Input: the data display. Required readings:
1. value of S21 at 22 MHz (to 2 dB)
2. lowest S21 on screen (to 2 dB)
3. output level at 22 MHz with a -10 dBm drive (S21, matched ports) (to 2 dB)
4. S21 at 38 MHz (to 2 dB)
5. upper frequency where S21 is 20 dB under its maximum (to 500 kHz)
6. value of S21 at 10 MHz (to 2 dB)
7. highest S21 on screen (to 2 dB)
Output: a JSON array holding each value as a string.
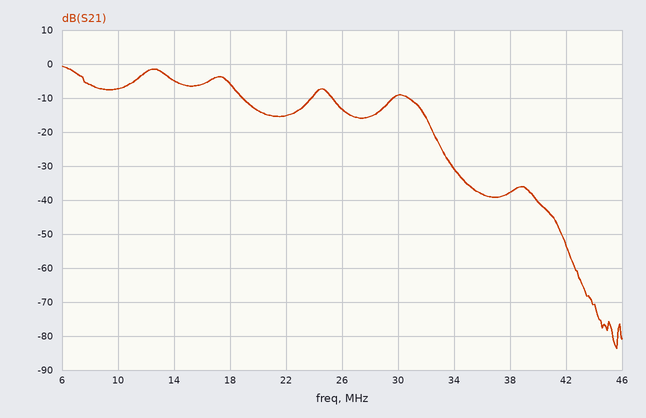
["-16 dB", "-84 dB", "-26 dBm", "-38 dB", "32.5 MHz", "-8 dB", "0 dB"]
